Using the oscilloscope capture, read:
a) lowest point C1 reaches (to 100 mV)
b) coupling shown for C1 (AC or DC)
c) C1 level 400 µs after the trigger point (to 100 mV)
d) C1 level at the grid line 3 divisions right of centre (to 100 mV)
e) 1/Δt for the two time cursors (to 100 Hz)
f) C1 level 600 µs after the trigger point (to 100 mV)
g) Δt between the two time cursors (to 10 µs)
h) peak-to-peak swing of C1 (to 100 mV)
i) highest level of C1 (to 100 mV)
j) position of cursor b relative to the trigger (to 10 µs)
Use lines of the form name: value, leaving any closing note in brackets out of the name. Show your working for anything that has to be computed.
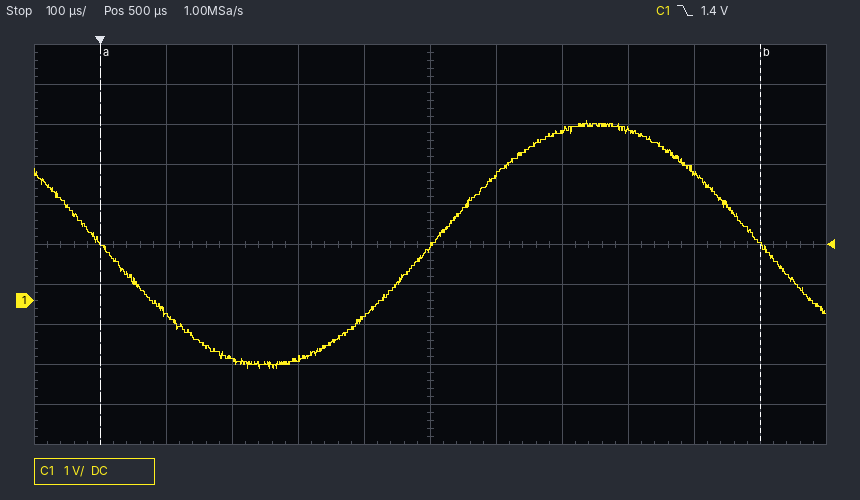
lowest point C1 reaches: -1.7 V
coupling shown for C1: DC
C1 level 400 µs after the trigger point: -400 mV
C1 level at the grid line 3 divisions right of centre: 4.3 V
1/Δt for the two time cursors: 1 / 1.00 ms ≈ 1.0 kHz
C1 level 600 µs after the trigger point: 3.1 V
Δt between the two time cursors: 1.00 ms
peak-to-peak swing of C1: 4.5 V − (-1.7 V) = 6.2 V
highest level of C1: 4.5 V
position of cursor b relative to the trigger: +1.00 ms
